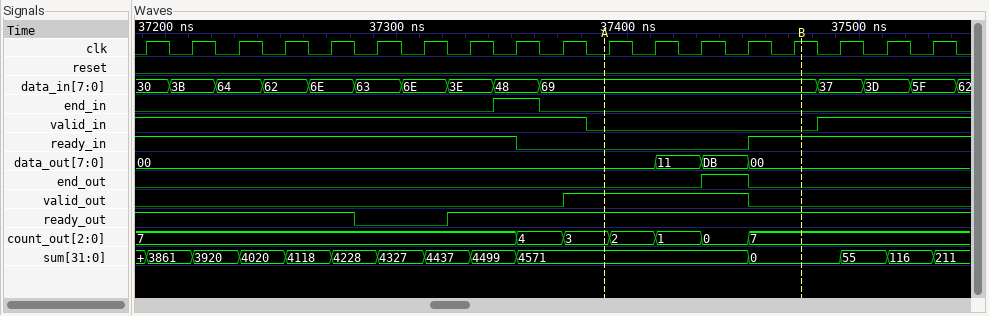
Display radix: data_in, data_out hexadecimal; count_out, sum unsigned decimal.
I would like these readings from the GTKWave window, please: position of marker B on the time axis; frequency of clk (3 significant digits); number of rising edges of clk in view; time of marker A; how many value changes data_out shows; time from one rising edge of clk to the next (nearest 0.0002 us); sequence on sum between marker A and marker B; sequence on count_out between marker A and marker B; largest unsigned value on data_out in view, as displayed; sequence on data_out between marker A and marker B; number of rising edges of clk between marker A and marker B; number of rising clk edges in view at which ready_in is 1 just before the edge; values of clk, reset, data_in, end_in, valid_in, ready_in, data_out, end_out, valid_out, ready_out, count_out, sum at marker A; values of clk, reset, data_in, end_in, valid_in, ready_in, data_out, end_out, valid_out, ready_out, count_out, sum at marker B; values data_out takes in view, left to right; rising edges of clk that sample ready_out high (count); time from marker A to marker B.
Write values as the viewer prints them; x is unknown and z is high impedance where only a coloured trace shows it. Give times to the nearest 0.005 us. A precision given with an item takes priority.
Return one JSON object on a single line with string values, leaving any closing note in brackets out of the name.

{"position of marker B on the time axis": "37.475 us", "frequency of clk": "50.0 MHz", "number of rising edges of clk in view": "18", "time of marker A": "37.39 us", "how many value changes data_out shows": "3", "time from one rising edge of clk to the next": "0.02 us", "sequence on sum between marker A and marker B": "4571, 0", "sequence on count_out between marker A and marker B": "3, 2, 1, 0, 7", "largest unsigned value on data_out in view, as displayed": "DB", "sequence on data_out between marker A and marker B": "00, 11, DB, 00", "number of rising edges of clk between marker A and marker B": "5", "number of rising clk edges in view at which ready_in is 1 just before the edge": "13", "values of clk, reset, data_in, end_in, valid_in, ready_in, data_out, end_out, valid_out, ready_out, count_out, sum at marker A": "clk=0, reset=0, data_in=69, end_in=0, valid_in=0, ready_in=0, data_out=00, end_out=0, valid_out=1, ready_out=1, count_out=3, sum=4571", "values of clk, reset, data_in, end_in, valid_in, ready_in, data_out, end_out, valid_out, ready_out, count_out, sum at marker B": "clk=1, reset=0, data_in=69, end_in=0, valid_in=0, ready_in=1, data_out=00, end_out=0, valid_out=0, ready_out=1, count_out=7, sum=0", "values data_out takes in view, left to right": "00, 11, DB, 00", "rising edges of clk that sample ready_out high": "16", "time from marker A to marker B": "0.085 us"}
